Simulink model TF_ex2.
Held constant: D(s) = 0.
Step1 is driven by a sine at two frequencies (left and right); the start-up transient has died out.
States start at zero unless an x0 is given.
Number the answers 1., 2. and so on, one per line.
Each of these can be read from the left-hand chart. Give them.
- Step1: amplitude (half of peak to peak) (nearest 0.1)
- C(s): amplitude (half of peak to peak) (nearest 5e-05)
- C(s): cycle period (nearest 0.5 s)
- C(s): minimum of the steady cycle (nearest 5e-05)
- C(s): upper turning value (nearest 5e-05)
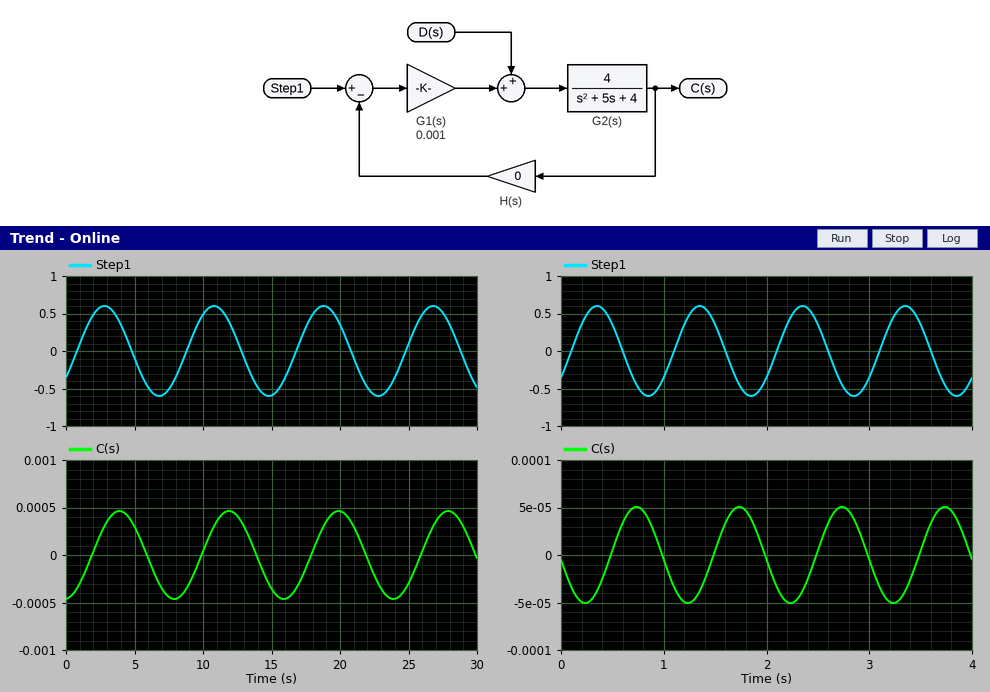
1. 0.6
2. 0.00045
3. 8.0 s
4. -0.00045
5. 0.00045
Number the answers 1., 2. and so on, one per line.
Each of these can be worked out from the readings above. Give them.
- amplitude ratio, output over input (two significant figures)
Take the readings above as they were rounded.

1. 0.00075
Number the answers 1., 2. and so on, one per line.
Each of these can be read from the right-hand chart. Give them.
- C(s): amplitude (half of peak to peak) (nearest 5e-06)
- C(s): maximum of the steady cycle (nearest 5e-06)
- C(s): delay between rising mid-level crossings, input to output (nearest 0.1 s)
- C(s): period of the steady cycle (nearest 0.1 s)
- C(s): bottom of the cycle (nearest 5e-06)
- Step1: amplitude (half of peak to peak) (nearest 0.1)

1. 0.000050
2. 0.000050
3. 0.4 s
4. 1.0 s
5. -0.000050
6. 0.6
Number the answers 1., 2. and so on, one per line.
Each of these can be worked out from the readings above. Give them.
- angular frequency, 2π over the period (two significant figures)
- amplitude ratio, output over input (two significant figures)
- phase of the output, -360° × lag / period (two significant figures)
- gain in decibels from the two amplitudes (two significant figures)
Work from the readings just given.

1. 6.3 rad/s
2. 0.000083
3. -140°
4. -82 dB
